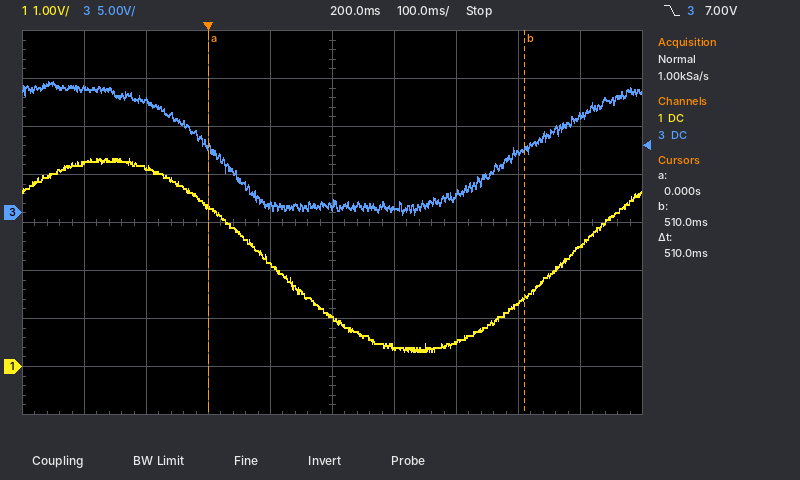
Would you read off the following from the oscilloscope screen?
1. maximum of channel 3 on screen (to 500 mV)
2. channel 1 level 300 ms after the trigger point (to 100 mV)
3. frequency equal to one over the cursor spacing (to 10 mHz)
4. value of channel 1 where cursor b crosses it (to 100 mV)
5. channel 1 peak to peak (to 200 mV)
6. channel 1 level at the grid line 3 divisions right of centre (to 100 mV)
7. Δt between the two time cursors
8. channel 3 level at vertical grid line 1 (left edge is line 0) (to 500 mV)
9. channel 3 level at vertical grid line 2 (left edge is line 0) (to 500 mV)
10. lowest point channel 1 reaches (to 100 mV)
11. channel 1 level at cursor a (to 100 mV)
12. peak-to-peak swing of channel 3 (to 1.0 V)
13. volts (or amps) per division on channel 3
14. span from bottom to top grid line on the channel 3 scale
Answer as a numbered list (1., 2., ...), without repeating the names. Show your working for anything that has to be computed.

1. 13.5 V
2. 400 mV
3. 1 / 510 ms ≈ 1.96 Hz
4. 1.4 V
5. 4.0 V
6. 1.3 V
7. 510 ms
8. 13.0 V
9. 11.5 V
10. 300 mV
11. 3.3 V
12. 14.0 V
13. 5 V
14. 40 V
